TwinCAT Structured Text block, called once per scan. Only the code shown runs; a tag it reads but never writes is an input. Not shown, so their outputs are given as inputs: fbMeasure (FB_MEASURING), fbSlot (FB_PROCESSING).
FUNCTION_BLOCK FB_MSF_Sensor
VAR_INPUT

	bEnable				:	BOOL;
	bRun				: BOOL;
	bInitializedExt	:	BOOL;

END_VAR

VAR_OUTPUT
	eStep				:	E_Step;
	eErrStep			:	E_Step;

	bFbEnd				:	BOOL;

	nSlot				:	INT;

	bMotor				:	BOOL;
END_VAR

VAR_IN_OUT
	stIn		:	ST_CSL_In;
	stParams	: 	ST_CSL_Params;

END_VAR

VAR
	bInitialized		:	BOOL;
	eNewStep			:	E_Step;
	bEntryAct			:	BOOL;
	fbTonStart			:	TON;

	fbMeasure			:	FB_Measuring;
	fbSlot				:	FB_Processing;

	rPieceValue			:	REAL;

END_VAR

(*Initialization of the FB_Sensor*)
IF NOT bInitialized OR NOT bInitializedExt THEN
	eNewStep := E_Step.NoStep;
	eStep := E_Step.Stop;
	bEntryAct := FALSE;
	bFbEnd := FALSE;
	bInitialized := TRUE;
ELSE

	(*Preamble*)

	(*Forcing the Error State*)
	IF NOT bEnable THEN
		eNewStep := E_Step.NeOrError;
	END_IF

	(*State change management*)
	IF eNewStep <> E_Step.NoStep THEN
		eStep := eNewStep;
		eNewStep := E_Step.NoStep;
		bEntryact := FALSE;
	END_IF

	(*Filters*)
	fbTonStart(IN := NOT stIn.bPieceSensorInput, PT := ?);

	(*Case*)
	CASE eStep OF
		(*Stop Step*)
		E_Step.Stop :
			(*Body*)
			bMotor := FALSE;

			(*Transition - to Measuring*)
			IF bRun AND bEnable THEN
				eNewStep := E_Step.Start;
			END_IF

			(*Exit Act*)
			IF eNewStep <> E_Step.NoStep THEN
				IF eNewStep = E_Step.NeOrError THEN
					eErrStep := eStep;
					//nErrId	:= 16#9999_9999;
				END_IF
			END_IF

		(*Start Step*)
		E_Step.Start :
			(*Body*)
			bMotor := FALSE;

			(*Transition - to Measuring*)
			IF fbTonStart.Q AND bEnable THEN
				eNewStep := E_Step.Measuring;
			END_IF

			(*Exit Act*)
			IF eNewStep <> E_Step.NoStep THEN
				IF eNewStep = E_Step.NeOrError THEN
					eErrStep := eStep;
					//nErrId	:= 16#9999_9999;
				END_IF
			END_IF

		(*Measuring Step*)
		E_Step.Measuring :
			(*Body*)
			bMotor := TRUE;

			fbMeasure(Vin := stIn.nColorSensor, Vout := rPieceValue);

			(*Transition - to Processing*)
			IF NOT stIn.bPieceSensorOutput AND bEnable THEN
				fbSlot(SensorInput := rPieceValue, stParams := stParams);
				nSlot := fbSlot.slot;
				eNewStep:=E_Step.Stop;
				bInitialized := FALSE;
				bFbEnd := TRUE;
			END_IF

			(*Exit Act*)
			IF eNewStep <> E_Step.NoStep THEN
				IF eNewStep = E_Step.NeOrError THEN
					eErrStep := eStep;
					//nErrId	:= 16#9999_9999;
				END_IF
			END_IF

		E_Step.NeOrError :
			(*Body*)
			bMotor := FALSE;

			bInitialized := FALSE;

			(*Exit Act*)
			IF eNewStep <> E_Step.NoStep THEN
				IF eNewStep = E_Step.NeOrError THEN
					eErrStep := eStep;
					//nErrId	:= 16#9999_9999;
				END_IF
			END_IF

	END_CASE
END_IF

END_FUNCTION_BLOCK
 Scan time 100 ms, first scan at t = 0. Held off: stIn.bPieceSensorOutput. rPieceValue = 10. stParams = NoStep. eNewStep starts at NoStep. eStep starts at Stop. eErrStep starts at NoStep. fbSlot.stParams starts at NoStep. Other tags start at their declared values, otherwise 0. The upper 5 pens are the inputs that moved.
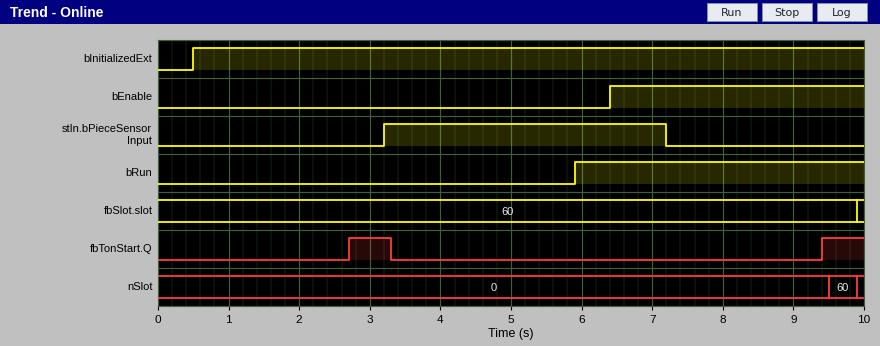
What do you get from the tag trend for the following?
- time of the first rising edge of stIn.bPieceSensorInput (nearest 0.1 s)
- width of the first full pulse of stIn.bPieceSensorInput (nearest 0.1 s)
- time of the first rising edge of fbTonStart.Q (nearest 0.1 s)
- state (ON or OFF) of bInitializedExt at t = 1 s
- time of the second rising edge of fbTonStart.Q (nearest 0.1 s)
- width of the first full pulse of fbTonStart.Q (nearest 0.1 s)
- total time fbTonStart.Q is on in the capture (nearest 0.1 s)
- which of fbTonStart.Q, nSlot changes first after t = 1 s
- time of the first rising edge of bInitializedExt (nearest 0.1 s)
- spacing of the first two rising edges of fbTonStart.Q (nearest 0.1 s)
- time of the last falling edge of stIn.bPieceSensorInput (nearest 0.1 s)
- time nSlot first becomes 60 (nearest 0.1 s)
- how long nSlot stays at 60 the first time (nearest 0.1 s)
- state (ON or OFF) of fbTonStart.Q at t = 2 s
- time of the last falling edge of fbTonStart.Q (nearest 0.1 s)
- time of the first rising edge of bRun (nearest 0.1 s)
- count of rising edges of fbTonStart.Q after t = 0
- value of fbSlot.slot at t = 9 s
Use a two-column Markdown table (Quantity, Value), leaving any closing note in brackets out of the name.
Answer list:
| Quantity | Value |
|---|---|
| time of the first rising edge of stIn.bPieceSensorInput | 3.2 s |
| width of the first full pulse of stIn.bPieceSensorInput | 4.0 s |
| time of the first rising edge of fbTonStart.Q | 2.7 s |
| state (ON or OFF) of bInitializedExt at t = 1 s | ON |
| time of the second rising edge of fbTonStart.Q | 9.4 s |
| width of the first full pulse of fbTonStart.Q | 0.6 s |
| total time fbTonStart.Q is on in the capture | 1.2 s |
| which of fbTonStart.Q, nSlot changes first after t = 1 s | fbTonStart.Q |
| time of the first rising edge of bInitializedExt | 0.5 s |
| spacing of the first two rising edges of fbTonStart.Q | 6.7 s |
| time of the last falling edge of stIn.bPieceSensorInput | 7.2 s |
| time nSlot first becomes 60 | 9.5 s |
| how long nSlot stays at 60 the first time | 0.4 s |
| state (ON or OFF) of fbTonStart.Q at t = 2 s | OFF |
| time of the last falling edge of fbTonStart.Q | 3.3 s |
| time of the first rising edge of bRun | 5.9 s |
| count of rising edges of fbTonStart.Q after t = 0 | 2 |
| value of fbSlot.slot at t = 9 s | 60 |
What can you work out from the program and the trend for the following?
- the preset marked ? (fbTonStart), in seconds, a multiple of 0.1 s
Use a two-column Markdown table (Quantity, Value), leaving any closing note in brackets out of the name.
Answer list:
| Quantity | Value |
|---|---|
| the preset marked ? (fbTonStart), in seconds, a multiple of 0.1 s | 2.2 s |
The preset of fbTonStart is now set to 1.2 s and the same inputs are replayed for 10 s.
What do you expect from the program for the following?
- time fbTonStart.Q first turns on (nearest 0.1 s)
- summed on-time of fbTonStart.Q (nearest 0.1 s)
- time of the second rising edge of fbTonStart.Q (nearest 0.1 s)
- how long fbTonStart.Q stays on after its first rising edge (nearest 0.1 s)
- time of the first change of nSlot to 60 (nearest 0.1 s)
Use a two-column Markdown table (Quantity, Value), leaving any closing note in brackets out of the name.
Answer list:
| Quantity | Value |
|---|---|
| time fbTonStart.Q first turns on | 1.7 s |
| summed on-time of fbTonStart.Q | 3.2 s |
| time of the second rising edge of fbTonStart.Q | 8.4 s |
| how long fbTonStart.Q stays on after its first rising edge | 1.6 s |
| time of the first change of nSlot to 60 | 8.5 s |
